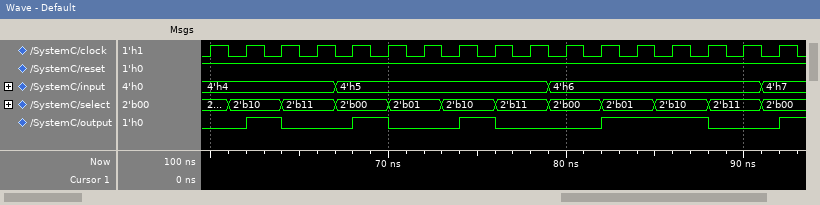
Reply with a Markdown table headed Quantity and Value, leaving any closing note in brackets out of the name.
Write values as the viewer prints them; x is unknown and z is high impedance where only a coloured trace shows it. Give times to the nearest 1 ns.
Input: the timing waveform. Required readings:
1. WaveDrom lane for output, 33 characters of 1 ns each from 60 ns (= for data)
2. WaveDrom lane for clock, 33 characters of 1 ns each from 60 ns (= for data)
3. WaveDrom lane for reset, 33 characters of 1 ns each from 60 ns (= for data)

| Quantity | Value |
|---|---|
| WaveDrom lane for output, 33 characters of 1 ns each from 60 ns | {name: 'output', wave: '0.1.0...1.0...1.0.....1.....0...1'} |
| WaveDrom lane for clock, 33 characters of 1 ns each from 60 ns | {name: 'clock', wave: '101010101010101010101010101010101'} |
| WaveDrom lane for reset, 33 characters of 1 ns each from 60 ns | {name: 'reset', wave: '1................................'} |
